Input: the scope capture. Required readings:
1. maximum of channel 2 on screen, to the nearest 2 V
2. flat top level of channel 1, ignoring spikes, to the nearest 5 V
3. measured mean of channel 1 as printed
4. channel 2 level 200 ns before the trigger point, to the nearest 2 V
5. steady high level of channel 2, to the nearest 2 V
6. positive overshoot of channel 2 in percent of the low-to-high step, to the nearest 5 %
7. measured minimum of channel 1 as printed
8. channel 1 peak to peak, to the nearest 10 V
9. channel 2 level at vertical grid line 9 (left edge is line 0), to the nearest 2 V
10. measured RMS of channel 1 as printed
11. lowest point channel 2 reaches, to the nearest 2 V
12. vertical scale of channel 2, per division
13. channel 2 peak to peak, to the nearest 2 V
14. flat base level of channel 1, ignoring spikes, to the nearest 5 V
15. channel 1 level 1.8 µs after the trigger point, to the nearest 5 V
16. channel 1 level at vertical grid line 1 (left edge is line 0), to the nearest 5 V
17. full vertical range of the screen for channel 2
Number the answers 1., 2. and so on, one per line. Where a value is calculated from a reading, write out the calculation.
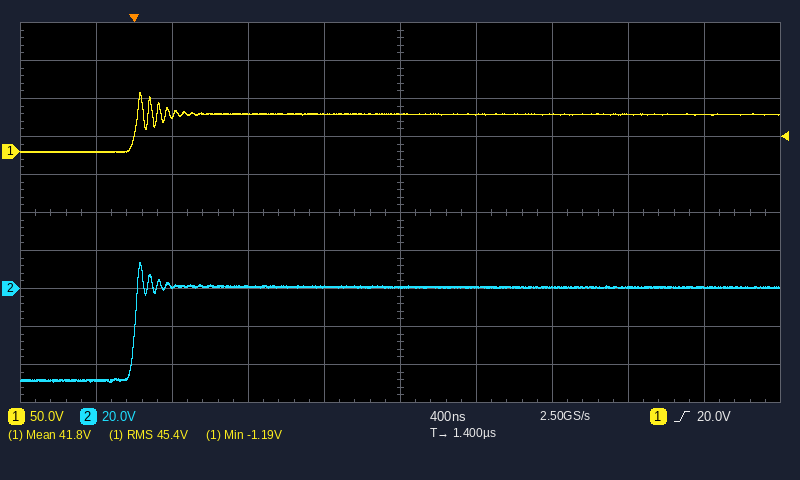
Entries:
1. 14 V
2. 50 V
3. 41.8 V
4. -48 V
5. 0 V
6. 25 %
7. -1.19 V
8. 80 V
9. 0 V
10. 45.4 V
11. -50 V
12. 20 V
13. 14 V − (-50 V) = 64 V
14. 0 V
15. 50 V
16. 0 V
17. 200 V
